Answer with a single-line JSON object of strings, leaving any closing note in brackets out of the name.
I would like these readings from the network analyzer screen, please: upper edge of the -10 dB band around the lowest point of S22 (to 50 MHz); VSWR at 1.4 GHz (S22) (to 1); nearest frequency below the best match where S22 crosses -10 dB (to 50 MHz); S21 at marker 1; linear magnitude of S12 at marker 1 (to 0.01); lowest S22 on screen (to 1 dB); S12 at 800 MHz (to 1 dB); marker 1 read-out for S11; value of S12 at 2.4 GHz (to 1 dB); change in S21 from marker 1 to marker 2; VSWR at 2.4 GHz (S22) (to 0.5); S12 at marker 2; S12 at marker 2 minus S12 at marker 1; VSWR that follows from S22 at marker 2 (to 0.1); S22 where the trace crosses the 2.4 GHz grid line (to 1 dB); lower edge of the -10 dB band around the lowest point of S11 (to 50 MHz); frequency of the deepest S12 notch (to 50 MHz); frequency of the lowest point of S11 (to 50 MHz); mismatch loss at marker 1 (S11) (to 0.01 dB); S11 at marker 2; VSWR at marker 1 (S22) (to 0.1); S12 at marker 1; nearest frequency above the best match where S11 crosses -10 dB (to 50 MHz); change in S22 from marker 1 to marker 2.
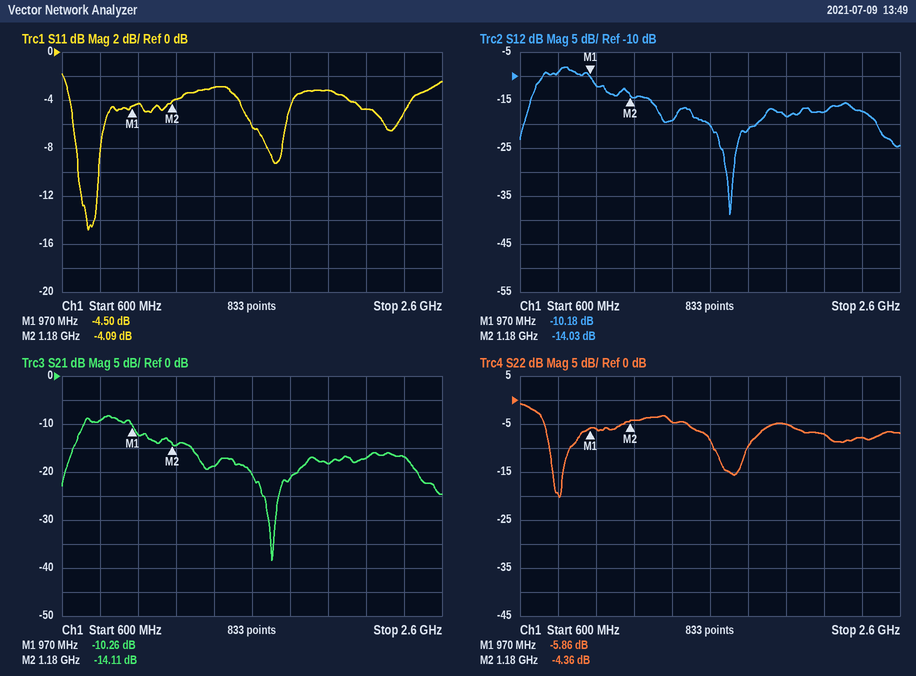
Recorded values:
{"upper edge of the -10 dB band around the lowest point of S22": "850 MHz", "VSWR at 1.4 GHz (S22)": "4", "nearest frequency below the best match where S22 crosses -10 dB": "750 MHz", "S21 at marker 1": "-10.26 dB", "linear magnitude of S12 at marker 1": "0.31", "lowest S22 on screen": "-20 dB", "S12 at 800 MHz": "-9 dB", "marker 1 read-out for S11": "-4.50 dB", "value of S12 at 2.4 GHz": "-17 dB", "change in S21 from marker 1 to marker 2": "-3.85 dB", "VSWR at 2.4 GHz (S22)": "2.5", "S12 at marker 2": "-14.03 dB", "S12 at marker 2 minus S12 at marker 1": "-3.85 dB", "VSWR that follows from S22 at marker 2": "4.1", "S22 where the trace crosses the 2.4 GHz grid line": "-8 dB", "lower edge of the -10 dB band around the lowest point of S11": "700 MHz", "frequency of the deepest S12 notch": "1.70 GHz", "frequency of the lowest point of S11": "750 MHz", "mismatch loss at marker 1 (S11)": "1.90 dB", "S11 at marker 2": "-4.09 dB", "VSWR at marker 1 (S22)": "3.1", "S12 at marker 1": "-10.18 dB", "nearest frequency above the best match where S11 crosses -10 dB": "800 MHz", "change in S22 from marker 1 to marker 2": "1.50 dB"}
